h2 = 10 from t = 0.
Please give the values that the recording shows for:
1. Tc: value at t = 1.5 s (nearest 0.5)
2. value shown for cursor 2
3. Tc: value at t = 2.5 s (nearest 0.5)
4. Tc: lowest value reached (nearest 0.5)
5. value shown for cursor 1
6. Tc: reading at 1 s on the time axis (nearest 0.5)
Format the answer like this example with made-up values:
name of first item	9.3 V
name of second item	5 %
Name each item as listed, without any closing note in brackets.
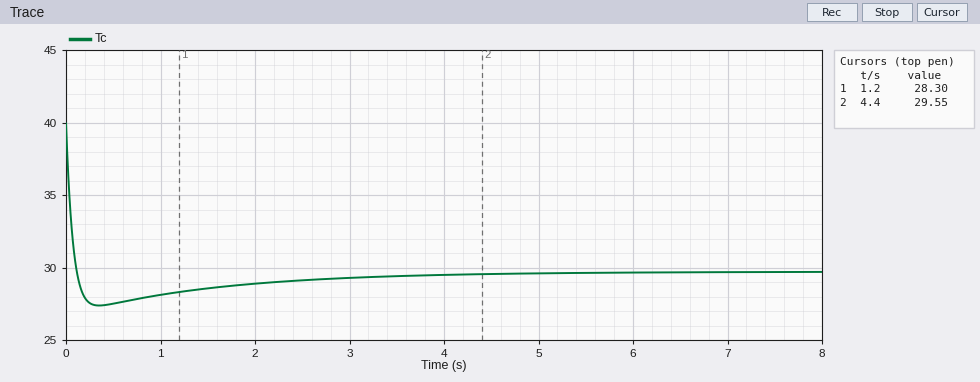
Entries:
Tc: value at t = 1.5 s	28.5
value shown for cursor 2	29.55
Tc: value at t = 2.5 s	29.0
Tc: lowest value reached	27.5
value shown for cursor 1	28.30
Tc: reading at 1 s on the time axis	28.0
